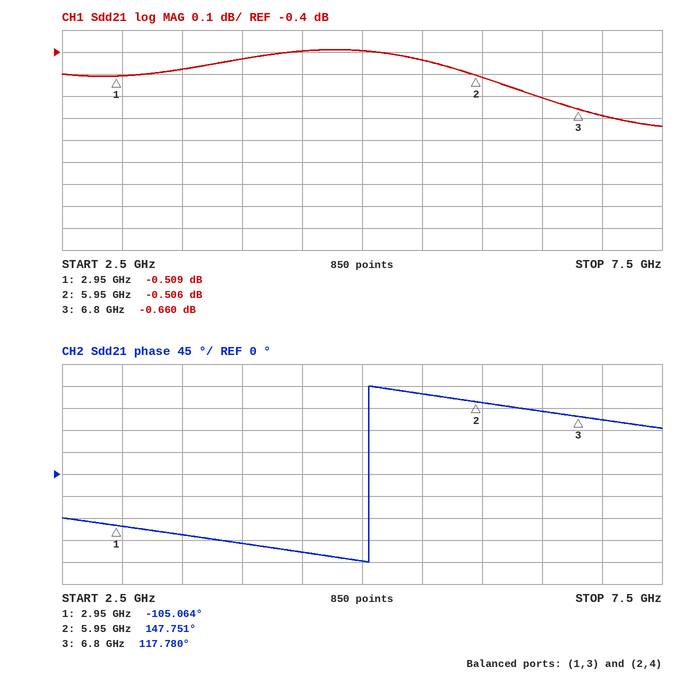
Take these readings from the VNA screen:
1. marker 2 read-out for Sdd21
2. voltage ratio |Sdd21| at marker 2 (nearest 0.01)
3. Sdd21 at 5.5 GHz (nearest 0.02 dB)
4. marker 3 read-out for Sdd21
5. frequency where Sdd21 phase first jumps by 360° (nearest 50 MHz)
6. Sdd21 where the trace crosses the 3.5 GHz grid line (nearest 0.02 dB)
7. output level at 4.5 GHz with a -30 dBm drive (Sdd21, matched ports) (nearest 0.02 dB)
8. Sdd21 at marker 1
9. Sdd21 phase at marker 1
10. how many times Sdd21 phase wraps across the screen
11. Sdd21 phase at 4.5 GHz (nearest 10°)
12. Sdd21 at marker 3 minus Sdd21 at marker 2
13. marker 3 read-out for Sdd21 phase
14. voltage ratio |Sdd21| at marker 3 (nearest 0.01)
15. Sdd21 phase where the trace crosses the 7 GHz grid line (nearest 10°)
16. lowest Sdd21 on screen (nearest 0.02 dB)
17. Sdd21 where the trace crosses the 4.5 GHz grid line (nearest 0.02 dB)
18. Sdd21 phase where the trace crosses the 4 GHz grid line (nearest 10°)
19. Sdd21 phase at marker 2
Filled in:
-0.506 dB
0.94
-0.44 dB
-0.660 dB
5.05 GHz
-0.48 dB
-30.40 dBm
-0.509 dB
-105.064°
1
-160°
-0.154 dB
117.780°
0.93
110°
-0.74 dB
-0.40 dB
-140°
147.751°
